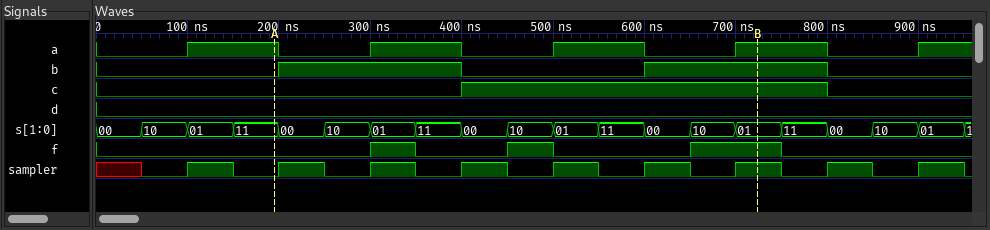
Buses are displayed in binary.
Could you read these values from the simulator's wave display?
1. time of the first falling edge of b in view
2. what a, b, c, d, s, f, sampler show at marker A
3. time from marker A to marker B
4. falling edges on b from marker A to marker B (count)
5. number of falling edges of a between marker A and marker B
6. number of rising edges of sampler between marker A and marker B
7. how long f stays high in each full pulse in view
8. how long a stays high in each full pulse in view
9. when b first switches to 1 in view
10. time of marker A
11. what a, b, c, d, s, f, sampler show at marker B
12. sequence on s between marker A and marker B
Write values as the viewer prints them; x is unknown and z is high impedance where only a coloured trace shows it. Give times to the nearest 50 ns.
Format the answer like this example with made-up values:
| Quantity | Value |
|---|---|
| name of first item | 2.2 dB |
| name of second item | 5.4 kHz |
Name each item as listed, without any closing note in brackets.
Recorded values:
| Quantity | Value |
|---|---|
| time of the first falling edge of b in view | 400 ns |
| what a, b, c, d, s, f, sampler show at marker A | a=1, b=0, c=0, d=0, s=11, f=0, sampler=0 |
| time from marker A to marker B | 550 ns |
| falling edges on b from marker A to marker B | 1 |
| number of falling edges of a between marker A and marker B | 3 |
| number of rising edges of sampler between marker A and marker B | 6 |
| how long f stays high in each full pulse in view | 50 ns, 50 ns, 100 ns |
| how long a stays high in each full pulse in view | 100 ns, 100 ns, 100 ns, 100 ns |
| when b first switches to 1 in view | 200 ns |
| time of marker A | 200 ns |
| what a, b, c, d, s, f, sampler show at marker B | a=1, b=1, c=1, d=0, s=01, f=1, sampler=1 |
| sequence on s between marker A and marker B | 11, 00, 10, 01, 11, 00, 10, 01, 11, 00, 10, 01 |
